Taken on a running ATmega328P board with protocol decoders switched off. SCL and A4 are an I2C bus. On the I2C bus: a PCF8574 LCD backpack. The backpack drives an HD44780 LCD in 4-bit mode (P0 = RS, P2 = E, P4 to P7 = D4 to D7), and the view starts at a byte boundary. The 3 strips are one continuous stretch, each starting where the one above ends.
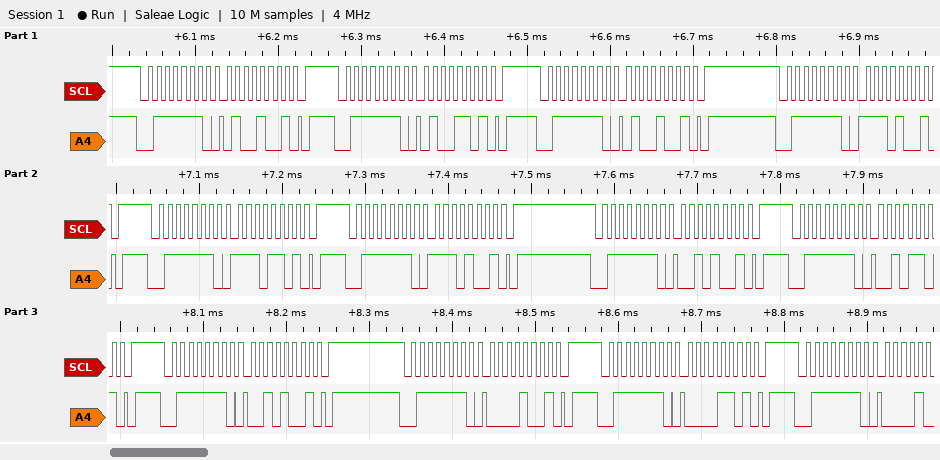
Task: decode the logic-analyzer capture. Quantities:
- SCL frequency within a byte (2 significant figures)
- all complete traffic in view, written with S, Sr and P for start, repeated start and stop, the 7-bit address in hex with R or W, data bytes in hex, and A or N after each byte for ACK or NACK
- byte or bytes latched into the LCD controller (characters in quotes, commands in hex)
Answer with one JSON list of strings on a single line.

["100 kHz", "S 3FW A 49 A P S 3FW A 4D A P S 3FW A 49 A P S 3FW A E9 A P S 3FW A ED A P S 3FW A E9 A P S 3FW A 29 A P S 3FW A 2D A P S 3FW A 29 A P S 3FW A 09 A P S 3FW A 0D A P S 3FW A", "'N'"]
